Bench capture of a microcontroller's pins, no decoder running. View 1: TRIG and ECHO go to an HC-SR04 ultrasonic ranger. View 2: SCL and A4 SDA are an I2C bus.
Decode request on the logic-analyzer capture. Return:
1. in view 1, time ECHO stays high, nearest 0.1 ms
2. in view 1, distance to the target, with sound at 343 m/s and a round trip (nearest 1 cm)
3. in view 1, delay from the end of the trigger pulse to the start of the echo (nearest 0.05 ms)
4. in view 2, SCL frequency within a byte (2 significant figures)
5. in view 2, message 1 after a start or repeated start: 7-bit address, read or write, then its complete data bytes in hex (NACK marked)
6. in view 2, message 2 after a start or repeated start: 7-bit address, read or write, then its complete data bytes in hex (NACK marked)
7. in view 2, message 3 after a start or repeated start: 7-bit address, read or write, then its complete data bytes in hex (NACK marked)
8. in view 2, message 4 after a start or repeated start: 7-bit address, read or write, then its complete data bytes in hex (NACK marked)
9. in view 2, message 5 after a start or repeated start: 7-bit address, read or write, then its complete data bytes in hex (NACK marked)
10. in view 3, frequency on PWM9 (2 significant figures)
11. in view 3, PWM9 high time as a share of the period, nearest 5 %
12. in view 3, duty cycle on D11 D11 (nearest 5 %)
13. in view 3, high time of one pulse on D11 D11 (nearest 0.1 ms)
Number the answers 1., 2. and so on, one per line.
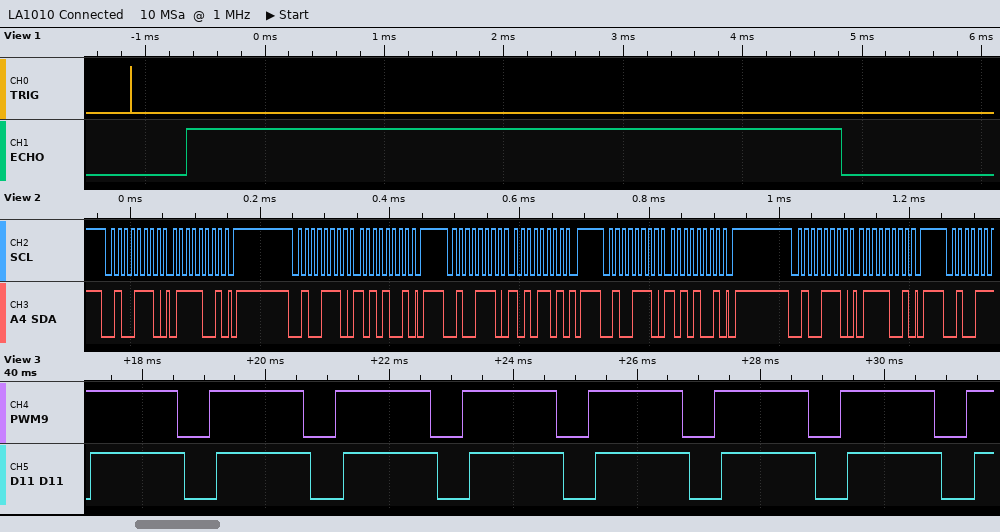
1. 5.5 ms
2. 94 cm
3. 0.45 ms
4. 100 kHz
5. 0x27 write: 79
6. 0x27 write: A9
7. 0x27 write: AD
8. 0x27 write: A9
9. 0x27 write: 79
10. 490 Hz
11. 75 %
12. 75 %
13. 1.5 ms
